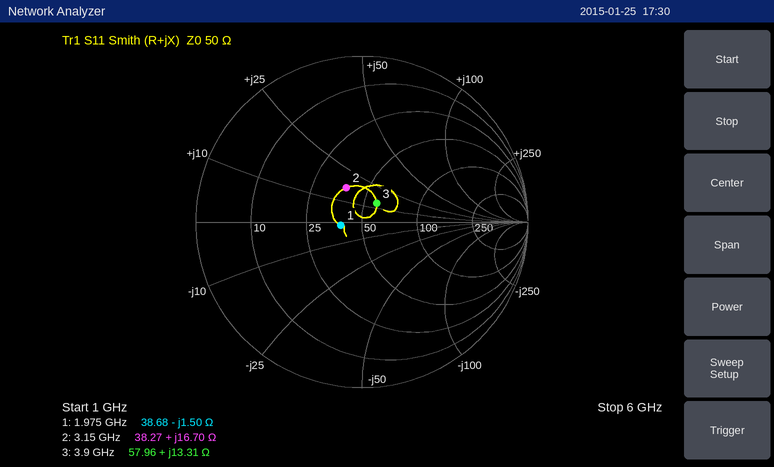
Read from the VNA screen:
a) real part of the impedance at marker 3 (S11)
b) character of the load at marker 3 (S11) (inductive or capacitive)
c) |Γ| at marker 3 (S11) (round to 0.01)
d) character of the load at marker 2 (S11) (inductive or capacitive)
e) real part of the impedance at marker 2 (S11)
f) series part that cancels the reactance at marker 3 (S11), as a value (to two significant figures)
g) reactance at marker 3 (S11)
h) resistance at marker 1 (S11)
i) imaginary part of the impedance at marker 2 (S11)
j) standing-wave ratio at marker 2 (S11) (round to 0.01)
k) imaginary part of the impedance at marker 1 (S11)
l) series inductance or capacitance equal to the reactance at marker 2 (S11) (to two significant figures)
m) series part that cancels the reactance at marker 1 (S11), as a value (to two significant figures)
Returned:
57.96 Ω
inductive
0.14
inductive
38.27 Ω
3.1 pF
+13.31 Ω
38.68 Ω
+16.70 Ω
1.59
-1.50 Ω
840 pH
120 pH
